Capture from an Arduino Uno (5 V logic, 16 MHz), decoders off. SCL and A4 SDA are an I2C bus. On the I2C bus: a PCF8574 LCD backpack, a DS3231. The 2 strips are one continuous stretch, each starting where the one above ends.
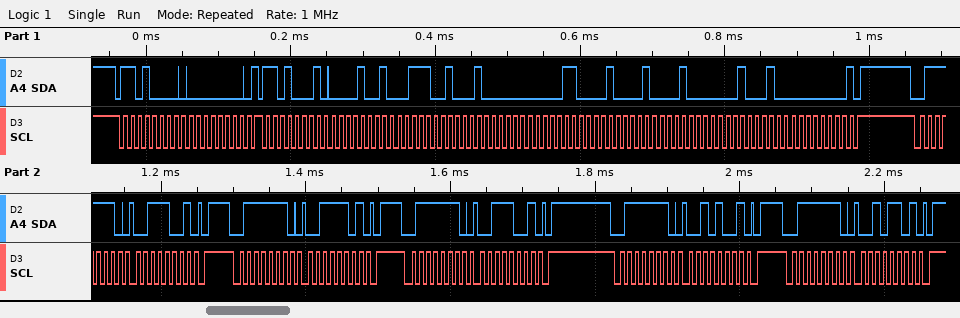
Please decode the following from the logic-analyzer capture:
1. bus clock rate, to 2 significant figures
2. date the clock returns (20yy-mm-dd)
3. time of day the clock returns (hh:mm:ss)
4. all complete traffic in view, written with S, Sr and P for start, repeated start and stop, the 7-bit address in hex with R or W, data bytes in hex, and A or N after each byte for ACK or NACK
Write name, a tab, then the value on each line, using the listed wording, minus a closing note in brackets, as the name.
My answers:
bus clock rate, to 2 significant figures	100 kHz
date the clock returns	2022-10-21
time of day the clock returns	20:39:09
all complete traffic in view, written with S, Sr and P for start, repeated start and stop, the 7-bit address in hex with R or W, data bytes in hex, and A or N after each byte for ACK or NACK	S 68W A 00 A Sr 68R A 09 A 39 A 20 A 06 A 21 A 10 A 22 A 00 N P S 3FW A 39 A P S 3FW A 3D A P S 3FW A 39 A P S 3FW A 29 A P S 3FW A 2D A P
